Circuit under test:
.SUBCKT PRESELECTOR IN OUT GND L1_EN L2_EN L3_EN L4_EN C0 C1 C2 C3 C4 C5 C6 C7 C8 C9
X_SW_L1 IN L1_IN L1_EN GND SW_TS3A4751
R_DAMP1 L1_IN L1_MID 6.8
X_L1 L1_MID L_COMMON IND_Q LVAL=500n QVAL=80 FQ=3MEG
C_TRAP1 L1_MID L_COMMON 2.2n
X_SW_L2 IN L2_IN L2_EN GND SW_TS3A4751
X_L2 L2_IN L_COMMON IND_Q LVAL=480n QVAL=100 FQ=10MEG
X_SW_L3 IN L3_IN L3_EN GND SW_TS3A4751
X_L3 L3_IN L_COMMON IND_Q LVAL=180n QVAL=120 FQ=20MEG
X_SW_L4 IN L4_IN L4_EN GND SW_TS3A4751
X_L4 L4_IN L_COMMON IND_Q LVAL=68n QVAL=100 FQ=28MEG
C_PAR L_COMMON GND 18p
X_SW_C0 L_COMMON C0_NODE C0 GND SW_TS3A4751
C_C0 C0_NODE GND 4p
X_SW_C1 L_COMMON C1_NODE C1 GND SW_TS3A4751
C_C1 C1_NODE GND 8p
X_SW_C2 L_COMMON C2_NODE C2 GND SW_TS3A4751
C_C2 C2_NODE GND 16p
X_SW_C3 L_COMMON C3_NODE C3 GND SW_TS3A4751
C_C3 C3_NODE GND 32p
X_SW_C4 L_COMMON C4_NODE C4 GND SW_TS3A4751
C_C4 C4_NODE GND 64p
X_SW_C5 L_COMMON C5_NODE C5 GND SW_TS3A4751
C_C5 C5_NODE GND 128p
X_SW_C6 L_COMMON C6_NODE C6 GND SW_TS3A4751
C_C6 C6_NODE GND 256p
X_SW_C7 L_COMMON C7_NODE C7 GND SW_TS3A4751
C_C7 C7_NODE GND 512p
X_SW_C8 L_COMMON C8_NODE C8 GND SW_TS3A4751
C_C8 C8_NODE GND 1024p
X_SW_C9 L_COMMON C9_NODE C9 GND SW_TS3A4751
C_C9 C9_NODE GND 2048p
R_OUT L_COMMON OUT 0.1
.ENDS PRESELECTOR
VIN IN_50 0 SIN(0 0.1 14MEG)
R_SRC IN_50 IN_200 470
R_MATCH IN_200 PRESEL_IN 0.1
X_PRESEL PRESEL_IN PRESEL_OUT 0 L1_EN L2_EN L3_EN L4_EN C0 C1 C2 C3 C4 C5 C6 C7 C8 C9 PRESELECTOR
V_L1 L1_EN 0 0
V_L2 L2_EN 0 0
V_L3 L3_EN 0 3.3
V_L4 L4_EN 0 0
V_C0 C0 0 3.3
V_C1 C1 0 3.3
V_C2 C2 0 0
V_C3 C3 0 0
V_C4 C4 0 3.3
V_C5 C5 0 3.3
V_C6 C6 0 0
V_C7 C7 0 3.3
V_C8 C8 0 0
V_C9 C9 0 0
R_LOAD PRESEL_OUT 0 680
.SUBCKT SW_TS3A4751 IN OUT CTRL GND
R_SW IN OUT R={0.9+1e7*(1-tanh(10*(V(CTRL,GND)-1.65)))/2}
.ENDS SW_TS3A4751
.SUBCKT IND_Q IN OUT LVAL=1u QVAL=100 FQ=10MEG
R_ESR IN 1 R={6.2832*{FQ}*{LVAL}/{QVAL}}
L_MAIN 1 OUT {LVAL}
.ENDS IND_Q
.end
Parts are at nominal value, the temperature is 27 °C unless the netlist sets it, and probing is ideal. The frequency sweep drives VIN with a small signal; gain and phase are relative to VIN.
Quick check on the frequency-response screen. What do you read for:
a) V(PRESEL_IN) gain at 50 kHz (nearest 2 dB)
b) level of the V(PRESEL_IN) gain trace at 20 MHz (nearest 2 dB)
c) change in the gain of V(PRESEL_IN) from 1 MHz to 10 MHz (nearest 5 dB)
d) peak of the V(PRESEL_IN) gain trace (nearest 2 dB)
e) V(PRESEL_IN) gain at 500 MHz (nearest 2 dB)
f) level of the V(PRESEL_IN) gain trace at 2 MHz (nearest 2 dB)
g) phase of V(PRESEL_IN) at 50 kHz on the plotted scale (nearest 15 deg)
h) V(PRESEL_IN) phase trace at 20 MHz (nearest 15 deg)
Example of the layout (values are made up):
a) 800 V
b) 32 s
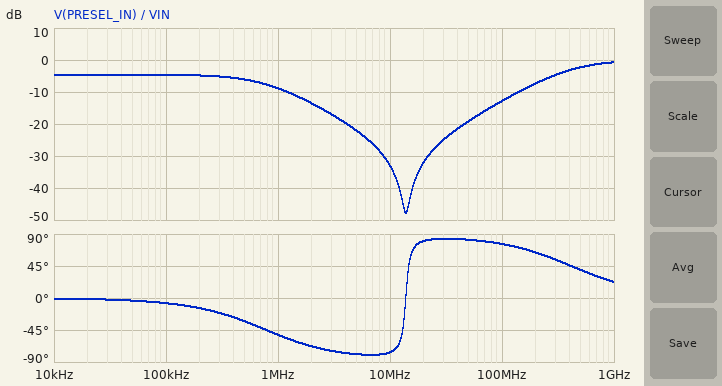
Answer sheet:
a) -4 dB
b) -32 dB
c) -25 dB
d) 0 dB
e) -2 dB
f) -14 dB
g) 0 deg
h) 75 deg
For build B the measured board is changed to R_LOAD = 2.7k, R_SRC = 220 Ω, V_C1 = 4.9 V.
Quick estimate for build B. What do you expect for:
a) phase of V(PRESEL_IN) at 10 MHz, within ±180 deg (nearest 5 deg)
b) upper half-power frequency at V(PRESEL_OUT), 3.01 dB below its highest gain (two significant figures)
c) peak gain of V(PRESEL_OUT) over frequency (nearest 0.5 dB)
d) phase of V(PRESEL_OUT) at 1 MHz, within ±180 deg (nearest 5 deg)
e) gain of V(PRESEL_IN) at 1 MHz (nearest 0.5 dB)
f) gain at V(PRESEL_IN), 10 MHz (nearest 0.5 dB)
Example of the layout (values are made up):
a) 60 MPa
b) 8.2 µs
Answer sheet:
a) -80 deg
b) 1.1 MHz
c) -0.5 dB
d) -45 deg
e) -3.5 dB
f) -26.5 dB
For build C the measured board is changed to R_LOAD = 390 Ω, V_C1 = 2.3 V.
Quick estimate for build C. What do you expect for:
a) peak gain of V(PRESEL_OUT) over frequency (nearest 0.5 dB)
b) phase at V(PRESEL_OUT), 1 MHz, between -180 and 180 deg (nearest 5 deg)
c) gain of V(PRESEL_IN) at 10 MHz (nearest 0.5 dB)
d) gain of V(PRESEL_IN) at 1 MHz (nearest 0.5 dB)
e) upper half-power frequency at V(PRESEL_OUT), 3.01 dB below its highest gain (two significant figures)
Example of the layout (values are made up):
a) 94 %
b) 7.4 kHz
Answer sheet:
a) -7.0 dB
b) -45 deg
c) -33.0 dB
d) -10.0 dB
e) 1.0 MHz
